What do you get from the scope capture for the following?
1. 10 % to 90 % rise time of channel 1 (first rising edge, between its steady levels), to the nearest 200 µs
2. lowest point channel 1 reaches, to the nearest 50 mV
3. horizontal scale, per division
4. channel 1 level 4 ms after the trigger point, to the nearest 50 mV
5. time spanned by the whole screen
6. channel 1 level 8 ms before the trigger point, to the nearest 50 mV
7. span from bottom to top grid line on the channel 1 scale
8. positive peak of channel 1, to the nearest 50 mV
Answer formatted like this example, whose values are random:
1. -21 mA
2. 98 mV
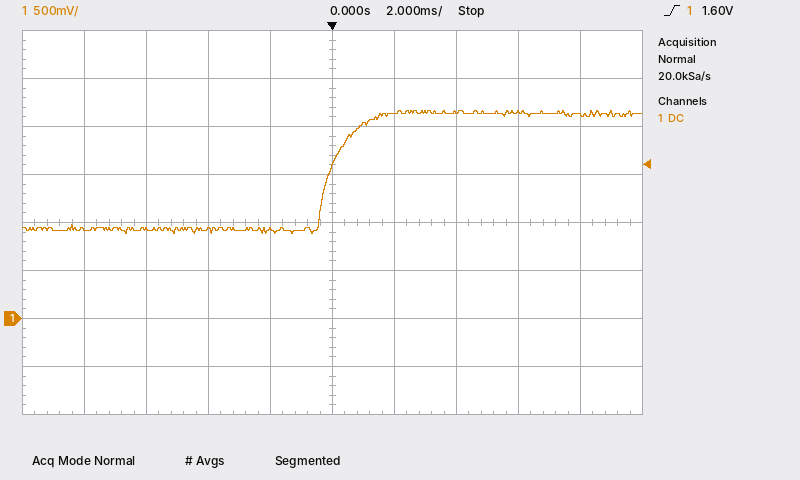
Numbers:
1. 1.4 ms
2. 900 mV
3. 2 ms
4. 2.15 V
5. 20 ms
6. 950 mV
7. 4 V
8. 2.15 V
